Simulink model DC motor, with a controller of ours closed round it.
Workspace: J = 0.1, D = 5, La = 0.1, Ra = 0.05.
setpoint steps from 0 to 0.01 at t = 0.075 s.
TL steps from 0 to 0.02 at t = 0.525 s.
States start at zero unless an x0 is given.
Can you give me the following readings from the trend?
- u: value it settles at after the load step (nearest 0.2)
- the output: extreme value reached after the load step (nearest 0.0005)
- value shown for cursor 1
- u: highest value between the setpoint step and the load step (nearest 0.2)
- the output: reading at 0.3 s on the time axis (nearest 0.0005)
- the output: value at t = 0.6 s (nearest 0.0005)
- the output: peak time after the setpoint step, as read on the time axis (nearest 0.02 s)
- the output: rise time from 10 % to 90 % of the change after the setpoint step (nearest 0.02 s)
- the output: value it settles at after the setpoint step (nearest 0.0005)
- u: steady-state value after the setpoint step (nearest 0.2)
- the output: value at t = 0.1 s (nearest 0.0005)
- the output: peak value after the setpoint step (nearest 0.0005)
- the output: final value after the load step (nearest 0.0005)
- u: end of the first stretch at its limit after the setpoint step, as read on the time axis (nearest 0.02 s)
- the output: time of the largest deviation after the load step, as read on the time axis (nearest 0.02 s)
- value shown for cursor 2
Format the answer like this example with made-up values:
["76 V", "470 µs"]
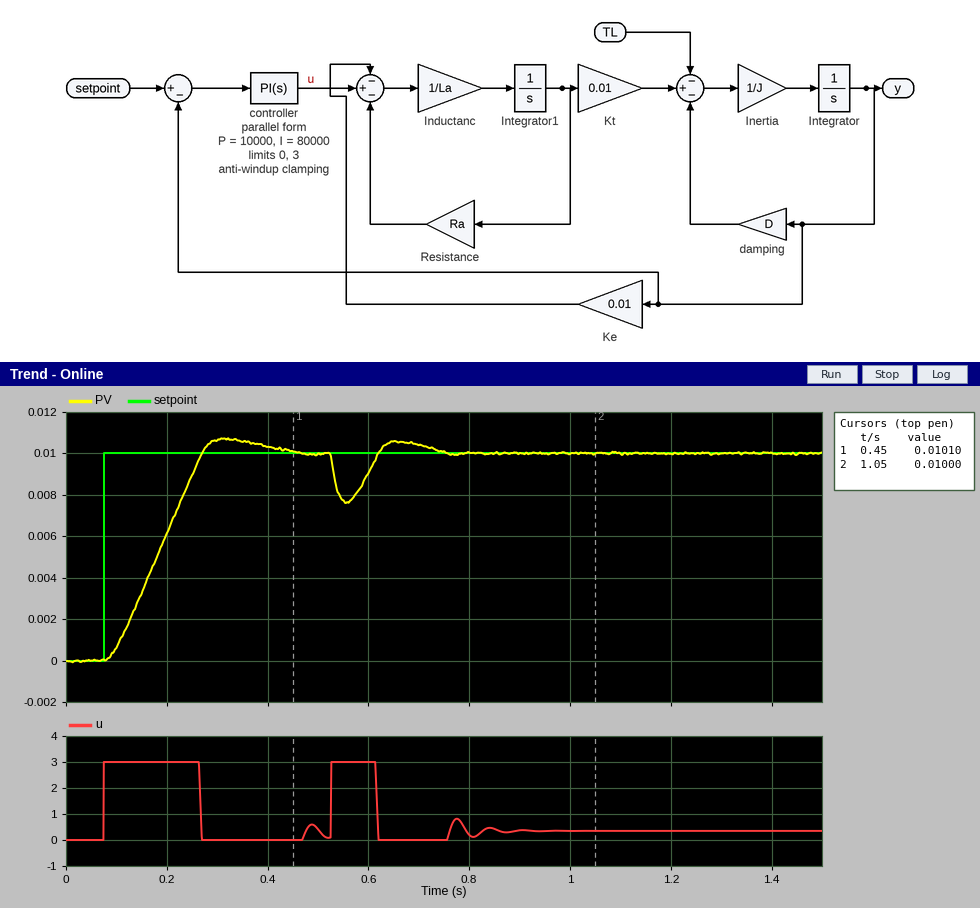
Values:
["0.4", "0.0075", "0.01010", "3.0", "0.0105", "0.0090", "0.32 s", "0.14 s", "0.0100", "0.2", "0.0005", "0.0105", "0.0100", "0.26 s", "0.56 s", "0.01000"]
